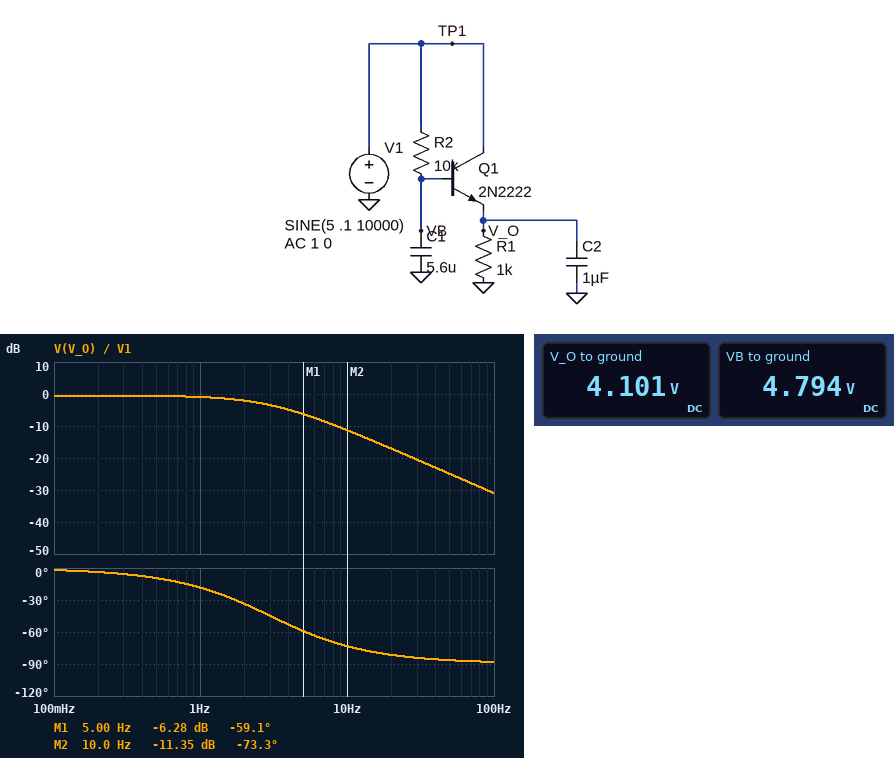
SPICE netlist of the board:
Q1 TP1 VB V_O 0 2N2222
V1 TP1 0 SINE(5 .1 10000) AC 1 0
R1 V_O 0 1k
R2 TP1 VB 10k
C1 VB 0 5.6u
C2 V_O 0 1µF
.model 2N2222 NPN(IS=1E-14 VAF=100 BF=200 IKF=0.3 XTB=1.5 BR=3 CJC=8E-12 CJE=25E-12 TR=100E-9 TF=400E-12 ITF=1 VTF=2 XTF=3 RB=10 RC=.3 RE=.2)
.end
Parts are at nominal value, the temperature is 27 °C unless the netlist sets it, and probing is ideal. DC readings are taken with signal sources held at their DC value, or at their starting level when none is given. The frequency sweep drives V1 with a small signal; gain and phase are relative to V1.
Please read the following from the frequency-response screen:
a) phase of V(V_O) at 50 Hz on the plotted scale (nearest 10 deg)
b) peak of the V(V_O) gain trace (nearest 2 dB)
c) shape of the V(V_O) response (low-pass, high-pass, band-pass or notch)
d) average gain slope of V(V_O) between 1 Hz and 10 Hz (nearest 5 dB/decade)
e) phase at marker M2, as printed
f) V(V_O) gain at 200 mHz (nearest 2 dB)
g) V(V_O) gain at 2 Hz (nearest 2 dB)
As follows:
-90 deg
0 dB
low-pass
-10 dB/decade
-73.3 deg
0 dB
-2 dB
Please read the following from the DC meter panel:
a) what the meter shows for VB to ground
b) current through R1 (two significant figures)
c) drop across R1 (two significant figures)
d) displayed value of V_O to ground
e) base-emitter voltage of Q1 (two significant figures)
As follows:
4.794 V
4.1 mA
4.1 V
4.101 V
690 mV
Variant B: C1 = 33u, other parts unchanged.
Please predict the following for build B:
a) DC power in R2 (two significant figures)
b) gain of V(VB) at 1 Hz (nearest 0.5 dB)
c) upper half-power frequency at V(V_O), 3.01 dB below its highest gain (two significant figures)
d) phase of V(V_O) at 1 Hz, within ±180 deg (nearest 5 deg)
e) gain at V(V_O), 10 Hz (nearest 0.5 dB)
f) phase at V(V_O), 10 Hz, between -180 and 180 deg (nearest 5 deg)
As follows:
4.3 µW
-7.5 dB
510 mHz
-65 deg
-26.5 dB
-85 deg
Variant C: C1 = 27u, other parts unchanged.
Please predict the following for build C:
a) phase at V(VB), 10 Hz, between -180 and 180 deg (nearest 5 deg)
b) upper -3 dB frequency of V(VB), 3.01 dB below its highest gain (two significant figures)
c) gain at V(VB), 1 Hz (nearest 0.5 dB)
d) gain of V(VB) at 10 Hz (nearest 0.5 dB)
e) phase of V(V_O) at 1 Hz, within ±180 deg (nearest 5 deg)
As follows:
-85 deg
620 mHz
-6.0 dB
-24.5 dB
-60 deg
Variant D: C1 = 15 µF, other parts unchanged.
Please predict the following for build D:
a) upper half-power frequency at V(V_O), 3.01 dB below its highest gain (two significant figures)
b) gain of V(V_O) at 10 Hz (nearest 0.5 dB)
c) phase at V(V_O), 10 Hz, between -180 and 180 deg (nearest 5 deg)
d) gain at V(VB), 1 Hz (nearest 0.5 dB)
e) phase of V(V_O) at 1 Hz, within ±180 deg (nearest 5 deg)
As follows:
1.1 Hz
-19.5 dB
-85 deg
-3.0 dB
-40 deg
